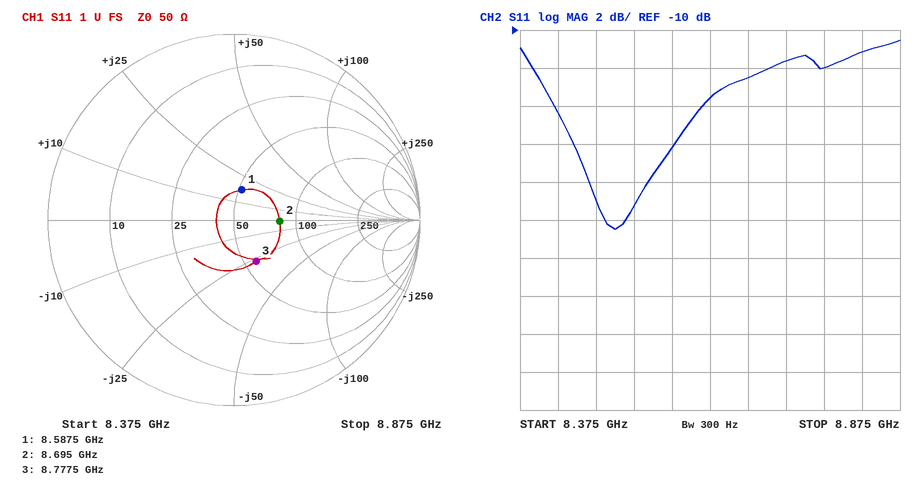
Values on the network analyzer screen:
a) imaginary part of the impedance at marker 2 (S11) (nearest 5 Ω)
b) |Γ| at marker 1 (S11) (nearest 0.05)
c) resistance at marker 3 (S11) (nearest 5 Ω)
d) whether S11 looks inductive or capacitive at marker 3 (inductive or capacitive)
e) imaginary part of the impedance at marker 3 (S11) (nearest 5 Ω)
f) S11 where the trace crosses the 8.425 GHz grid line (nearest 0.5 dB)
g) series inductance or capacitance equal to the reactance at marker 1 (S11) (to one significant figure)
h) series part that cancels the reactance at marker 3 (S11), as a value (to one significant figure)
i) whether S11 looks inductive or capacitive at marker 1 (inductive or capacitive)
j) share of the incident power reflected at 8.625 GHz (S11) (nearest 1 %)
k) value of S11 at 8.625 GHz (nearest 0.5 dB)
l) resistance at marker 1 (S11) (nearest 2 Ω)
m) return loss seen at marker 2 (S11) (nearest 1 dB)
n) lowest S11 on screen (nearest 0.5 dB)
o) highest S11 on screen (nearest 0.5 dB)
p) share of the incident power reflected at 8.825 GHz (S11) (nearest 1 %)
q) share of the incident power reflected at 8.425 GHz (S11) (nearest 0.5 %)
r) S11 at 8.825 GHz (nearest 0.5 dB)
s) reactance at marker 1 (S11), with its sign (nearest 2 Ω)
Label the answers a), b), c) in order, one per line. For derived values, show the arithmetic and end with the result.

a) 0 Ω
b) 0.15
c) 55 Ω
d) capacitive
e) -25 Ω
f) -14.5 dB
g) L = 18 Ω/(2π × 8.5875 GHz) ≈ 334 pH, so 300 pH to one significant figure
h) L = 25 Ω/(2π × 8.7775 GHz) ≈ 453 pH, so 500 pH to one significant figure
i) inductive
j) 10^(-13.5/10) ≈ 4 %
k) -13.5 dB
l) 52 Ω
m) 12 dB
n) -20.5 dB
o) -10.5 dB
p) 10^(-11/10) ≈ 8 %
q) 10^(-14.5/10) ≈ 3.5 %
r) -11.0 dB
s) +18 Ω
